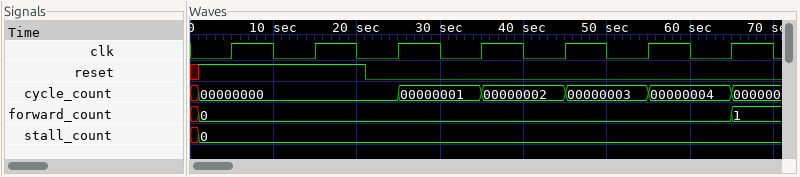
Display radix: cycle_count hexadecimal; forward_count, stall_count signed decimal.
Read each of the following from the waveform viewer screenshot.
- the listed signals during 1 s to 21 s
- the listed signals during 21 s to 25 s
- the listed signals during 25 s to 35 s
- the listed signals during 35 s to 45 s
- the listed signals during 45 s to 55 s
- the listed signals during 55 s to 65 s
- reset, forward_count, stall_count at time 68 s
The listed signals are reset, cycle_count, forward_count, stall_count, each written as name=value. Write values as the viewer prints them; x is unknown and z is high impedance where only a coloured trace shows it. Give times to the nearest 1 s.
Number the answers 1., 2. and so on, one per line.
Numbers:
1. reset=1, cycle_count=00000000, forward_count=0, stall_count=0
2. reset=0, cycle_count=00000000, forward_count=0, stall_count=0
3. reset=0, cycle_count=00000001, forward_count=0, stall_count=0
4. reset=0, cycle_count=00000002, forward_count=0, stall_count=0
5. reset=0, cycle_count=00000003, forward_count=0, stall_count=0
6. reset=0, cycle_count=00000004, forward_count=0, stall_count=0
7. reset=0, forward_count=1, stall_count=0
